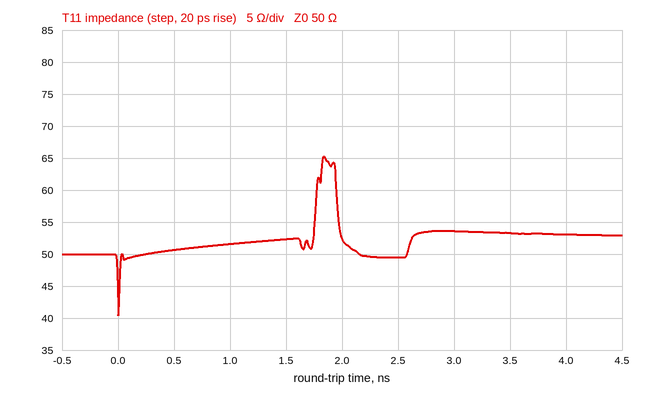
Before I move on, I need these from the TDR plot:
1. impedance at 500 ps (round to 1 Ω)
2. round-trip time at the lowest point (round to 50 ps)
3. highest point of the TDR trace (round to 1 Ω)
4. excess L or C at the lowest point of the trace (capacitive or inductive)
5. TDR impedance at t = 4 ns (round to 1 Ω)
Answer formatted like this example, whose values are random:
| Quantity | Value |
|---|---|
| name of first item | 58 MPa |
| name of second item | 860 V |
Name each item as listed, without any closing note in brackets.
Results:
| Quantity | Value |
|---|---|
| impedance at 500 ps | 51 Ω |
| round-trip time at the lowest point | 0 ps |
| highest point of the TDR trace | 65 Ω |
| excess L or C at the lowest point of the trace | capacitive |
| TDR impedance at t = 4 ns | 53 Ω |
